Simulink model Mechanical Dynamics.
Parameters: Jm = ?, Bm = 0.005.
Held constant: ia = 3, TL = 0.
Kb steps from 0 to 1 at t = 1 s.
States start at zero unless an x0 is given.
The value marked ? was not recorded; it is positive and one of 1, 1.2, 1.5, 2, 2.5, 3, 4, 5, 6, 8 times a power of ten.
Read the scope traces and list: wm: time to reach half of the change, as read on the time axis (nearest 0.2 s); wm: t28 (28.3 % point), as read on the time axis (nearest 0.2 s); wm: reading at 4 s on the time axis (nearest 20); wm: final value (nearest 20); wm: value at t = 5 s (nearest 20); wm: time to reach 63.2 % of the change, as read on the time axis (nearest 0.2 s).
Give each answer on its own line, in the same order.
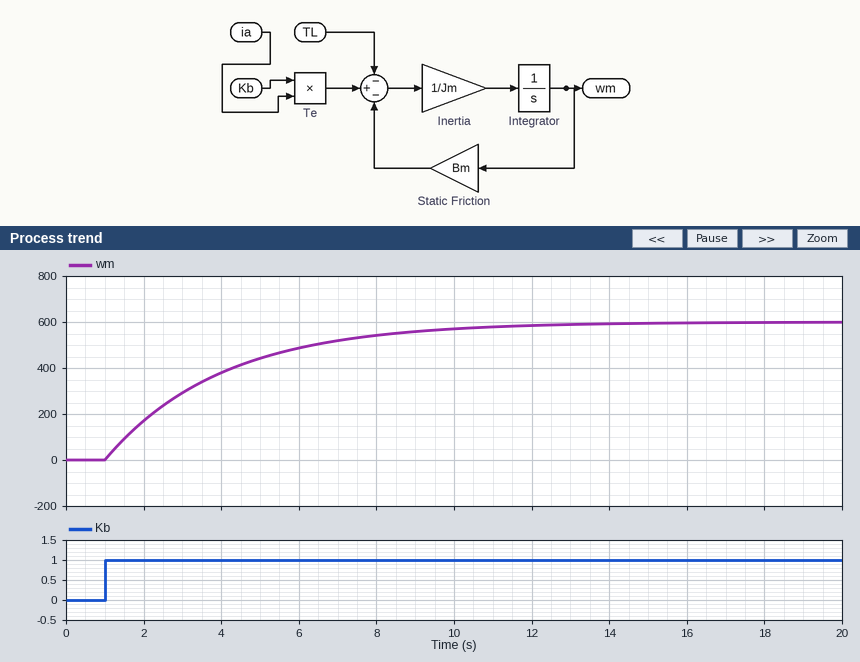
3.0 s
2.0 s
380
600
440
4.0 s
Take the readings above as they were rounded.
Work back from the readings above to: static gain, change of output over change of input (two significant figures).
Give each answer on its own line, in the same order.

600
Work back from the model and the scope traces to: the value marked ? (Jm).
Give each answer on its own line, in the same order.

0.015
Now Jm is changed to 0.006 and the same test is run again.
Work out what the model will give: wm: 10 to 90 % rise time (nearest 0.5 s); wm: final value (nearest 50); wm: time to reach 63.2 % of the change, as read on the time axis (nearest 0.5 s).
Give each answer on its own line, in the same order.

2.5 s
600
2.0 s
